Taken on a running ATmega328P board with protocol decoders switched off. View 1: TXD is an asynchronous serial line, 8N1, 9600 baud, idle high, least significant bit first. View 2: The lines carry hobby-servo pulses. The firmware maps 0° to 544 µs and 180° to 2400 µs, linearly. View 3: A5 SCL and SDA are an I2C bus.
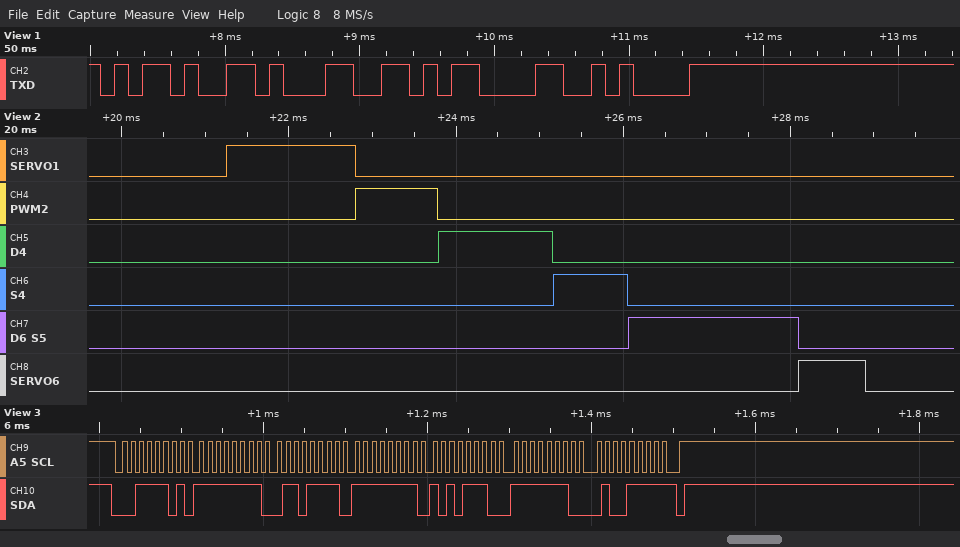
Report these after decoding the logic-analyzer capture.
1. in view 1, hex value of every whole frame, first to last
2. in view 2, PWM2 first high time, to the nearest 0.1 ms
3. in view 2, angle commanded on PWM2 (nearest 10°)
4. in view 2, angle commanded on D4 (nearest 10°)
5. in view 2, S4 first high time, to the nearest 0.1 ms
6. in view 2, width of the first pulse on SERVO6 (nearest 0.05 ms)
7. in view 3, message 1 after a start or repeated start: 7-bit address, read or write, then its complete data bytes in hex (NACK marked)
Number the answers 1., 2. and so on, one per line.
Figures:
1. 0x2D 0x31 0x0D 0x0A
2. 1.0 ms
3. 40°
4. 80°
5. 0.9 ms
6. 0.80 ms
7. 0x1E read: FF 6F FF AE FE 4F NACK
